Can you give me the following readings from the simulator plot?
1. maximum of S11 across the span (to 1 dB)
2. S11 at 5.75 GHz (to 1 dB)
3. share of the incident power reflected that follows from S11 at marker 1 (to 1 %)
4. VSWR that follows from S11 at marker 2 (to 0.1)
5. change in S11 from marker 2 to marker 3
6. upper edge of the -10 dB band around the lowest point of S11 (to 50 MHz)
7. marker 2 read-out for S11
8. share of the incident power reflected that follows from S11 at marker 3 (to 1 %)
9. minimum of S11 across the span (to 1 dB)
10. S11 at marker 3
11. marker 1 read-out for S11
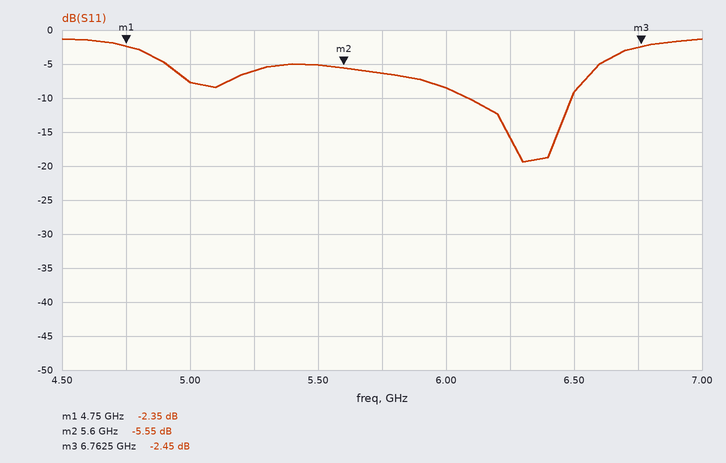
-1 dB
-6 dB
58 %
3.2
3.10 dB
6.50 GHz
-5.55 dB
57 %
-19 dB
-2.45 dB
-2.35 dB
